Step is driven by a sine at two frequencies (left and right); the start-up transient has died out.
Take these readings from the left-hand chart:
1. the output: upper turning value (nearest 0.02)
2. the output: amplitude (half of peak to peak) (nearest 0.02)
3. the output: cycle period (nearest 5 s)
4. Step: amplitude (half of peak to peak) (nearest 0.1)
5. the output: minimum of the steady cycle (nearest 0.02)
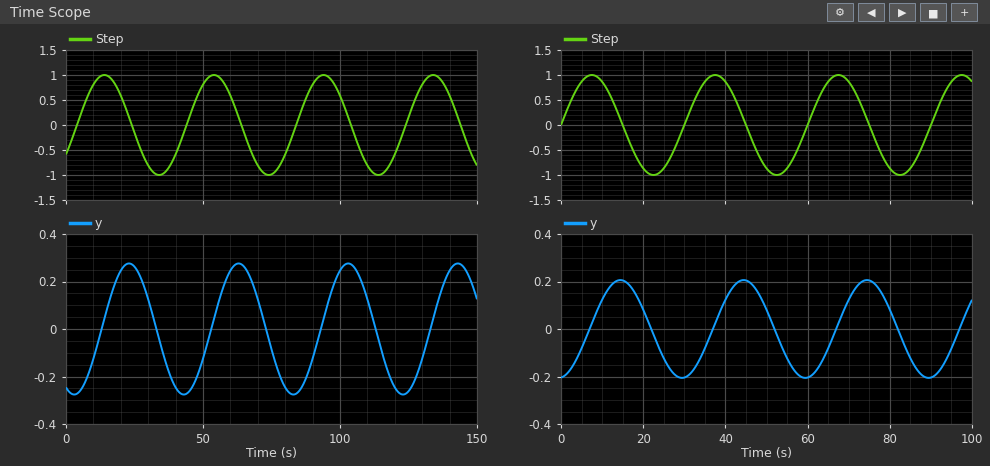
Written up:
0.28
0.28
40 s
1.0
-0.28
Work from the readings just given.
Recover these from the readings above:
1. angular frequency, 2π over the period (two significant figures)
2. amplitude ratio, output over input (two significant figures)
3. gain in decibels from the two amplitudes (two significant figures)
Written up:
0.16 rad/s
0.28
-11 dB
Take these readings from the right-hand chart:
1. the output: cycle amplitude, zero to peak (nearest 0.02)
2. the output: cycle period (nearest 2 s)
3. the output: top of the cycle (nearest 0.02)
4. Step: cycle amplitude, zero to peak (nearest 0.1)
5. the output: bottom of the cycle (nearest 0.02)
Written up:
0.20
30 s
0.20
1.0
-0.20
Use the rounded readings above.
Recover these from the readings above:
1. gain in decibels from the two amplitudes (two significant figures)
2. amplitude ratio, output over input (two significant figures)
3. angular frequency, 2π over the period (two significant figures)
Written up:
-14 dB
0.20
0.21 rad/s
